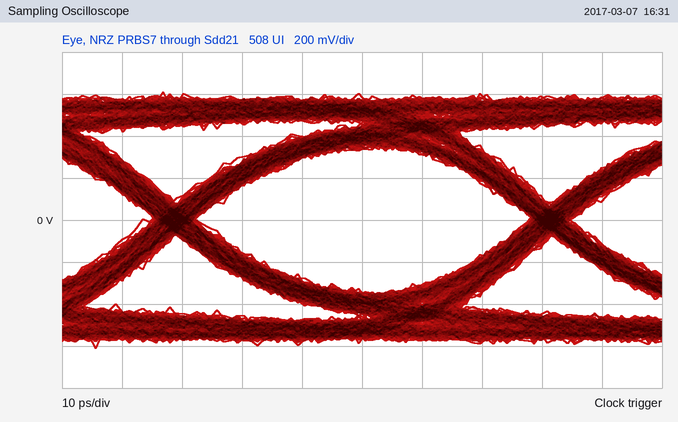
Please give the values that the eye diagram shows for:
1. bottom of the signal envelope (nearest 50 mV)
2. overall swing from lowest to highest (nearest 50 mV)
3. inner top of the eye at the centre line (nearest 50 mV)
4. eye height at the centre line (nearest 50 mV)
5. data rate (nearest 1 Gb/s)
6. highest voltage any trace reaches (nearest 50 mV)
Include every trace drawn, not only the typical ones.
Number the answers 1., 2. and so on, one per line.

1. -600 mV
2. 1.20 V
3. 350 mV
4. 700 mV
5. 16 Gb/s
6. 600 mV
